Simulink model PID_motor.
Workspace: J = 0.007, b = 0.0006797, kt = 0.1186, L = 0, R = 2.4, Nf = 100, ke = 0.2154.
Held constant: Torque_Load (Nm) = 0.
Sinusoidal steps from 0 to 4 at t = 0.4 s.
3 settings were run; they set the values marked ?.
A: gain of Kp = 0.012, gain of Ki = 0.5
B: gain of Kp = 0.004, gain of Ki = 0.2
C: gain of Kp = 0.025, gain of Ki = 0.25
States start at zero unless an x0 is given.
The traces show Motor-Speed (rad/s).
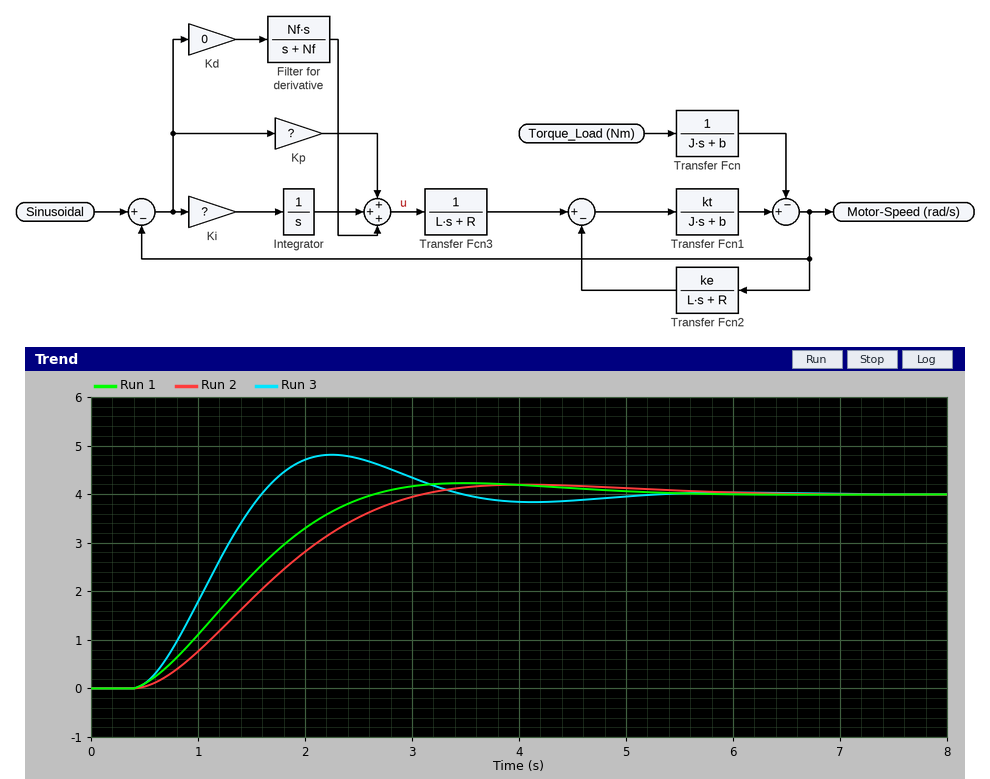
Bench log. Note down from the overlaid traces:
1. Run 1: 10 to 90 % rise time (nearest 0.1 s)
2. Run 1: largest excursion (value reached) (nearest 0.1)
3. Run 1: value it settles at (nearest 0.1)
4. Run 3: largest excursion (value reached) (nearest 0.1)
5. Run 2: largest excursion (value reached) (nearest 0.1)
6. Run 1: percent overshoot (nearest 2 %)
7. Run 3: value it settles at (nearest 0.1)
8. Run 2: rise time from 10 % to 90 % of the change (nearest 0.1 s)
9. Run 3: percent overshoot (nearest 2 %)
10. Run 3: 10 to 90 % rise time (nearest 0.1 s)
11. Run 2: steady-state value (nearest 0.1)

1.5 s
4.2
4.0
4.8
4.2
6 %
4.0
1.8 s
20 %
0.8 s
4.0
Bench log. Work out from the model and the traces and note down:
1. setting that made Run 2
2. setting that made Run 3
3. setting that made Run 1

B
A
C
